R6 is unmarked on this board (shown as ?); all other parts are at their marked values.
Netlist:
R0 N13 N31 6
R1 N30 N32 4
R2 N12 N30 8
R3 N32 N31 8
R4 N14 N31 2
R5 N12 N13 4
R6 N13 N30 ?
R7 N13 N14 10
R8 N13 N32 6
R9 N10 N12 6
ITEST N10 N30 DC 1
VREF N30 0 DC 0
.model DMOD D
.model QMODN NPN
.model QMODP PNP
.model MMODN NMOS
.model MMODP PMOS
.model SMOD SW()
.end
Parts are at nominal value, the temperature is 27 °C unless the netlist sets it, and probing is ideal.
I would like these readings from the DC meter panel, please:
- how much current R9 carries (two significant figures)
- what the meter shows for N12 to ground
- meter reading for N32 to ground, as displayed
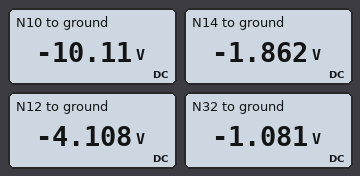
1.0 A
-4.108 V
-1.081 V
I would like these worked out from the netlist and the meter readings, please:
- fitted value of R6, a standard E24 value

10 Ω
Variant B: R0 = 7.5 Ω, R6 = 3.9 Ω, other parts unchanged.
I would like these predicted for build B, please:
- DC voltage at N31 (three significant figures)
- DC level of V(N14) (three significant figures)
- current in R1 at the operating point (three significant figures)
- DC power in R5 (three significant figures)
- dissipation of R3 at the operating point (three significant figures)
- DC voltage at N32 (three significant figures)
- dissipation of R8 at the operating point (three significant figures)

-1.17 V
-1.22 V
178 mA
1.20 W
26.4 mW
-713 mV
87.5 mW
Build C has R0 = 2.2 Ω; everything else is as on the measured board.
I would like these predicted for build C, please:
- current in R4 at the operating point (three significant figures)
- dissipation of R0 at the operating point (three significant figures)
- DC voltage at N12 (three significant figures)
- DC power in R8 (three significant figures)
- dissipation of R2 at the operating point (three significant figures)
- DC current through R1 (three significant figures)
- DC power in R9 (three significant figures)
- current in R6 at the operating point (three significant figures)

16.2 mA
17.1 mW
-4.09 V
176 mW
2.09 W
276 mA
6.00 W
213 mA
